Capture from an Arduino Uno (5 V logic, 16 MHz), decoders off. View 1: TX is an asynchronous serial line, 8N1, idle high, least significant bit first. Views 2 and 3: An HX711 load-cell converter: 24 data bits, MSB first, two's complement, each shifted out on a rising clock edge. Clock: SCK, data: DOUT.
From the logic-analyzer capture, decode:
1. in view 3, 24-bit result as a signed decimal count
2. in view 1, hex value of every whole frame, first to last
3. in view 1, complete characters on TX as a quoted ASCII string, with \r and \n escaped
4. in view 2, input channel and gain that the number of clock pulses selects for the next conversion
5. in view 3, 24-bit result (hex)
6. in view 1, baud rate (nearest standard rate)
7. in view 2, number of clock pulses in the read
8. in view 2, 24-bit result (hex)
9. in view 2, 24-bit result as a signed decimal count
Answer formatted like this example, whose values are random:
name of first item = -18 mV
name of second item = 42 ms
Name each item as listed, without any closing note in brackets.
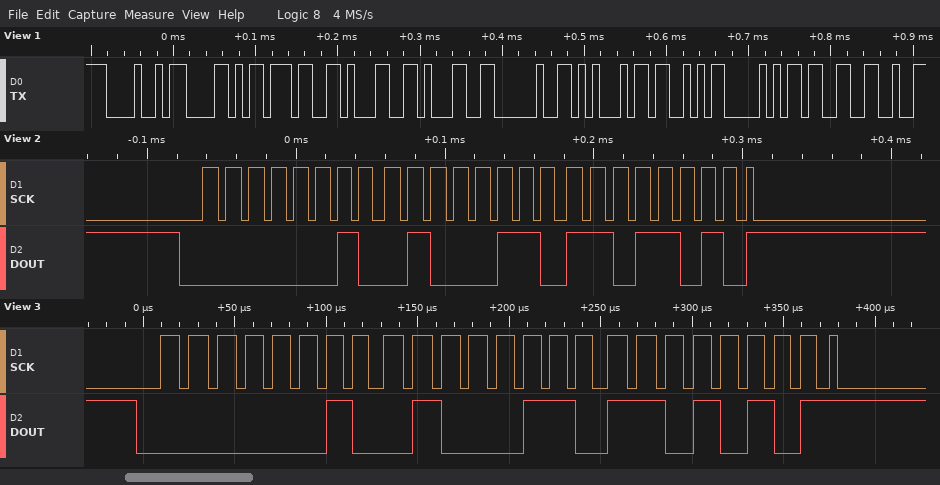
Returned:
in view 3, 24-bit result as a signed decimal count = 149205
in view 1, hex value of every whole frame, first to last = 48 58 37 31 31 20 45 53 50 33
in view 1, complete characters on TX as a quoted ASCII string, with \r and \n escaped = "HX711 ESP3"
in view 2, input channel and gain that the number of clock pulses selects for the next conversion = channel A, gain 128
in view 3, 24-bit result = 0x0246D5
in view 1, baud rate = 115200 baud
in view 2, number of clock pulses in the read = 25
in view 2, 24-bit result = 0x0246DA
in view 2, 24-bit result as a signed decimal count = 149210
